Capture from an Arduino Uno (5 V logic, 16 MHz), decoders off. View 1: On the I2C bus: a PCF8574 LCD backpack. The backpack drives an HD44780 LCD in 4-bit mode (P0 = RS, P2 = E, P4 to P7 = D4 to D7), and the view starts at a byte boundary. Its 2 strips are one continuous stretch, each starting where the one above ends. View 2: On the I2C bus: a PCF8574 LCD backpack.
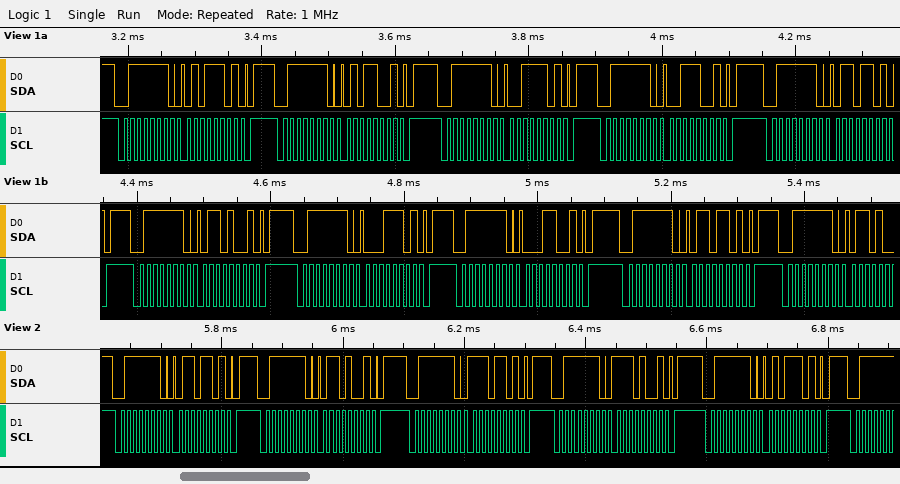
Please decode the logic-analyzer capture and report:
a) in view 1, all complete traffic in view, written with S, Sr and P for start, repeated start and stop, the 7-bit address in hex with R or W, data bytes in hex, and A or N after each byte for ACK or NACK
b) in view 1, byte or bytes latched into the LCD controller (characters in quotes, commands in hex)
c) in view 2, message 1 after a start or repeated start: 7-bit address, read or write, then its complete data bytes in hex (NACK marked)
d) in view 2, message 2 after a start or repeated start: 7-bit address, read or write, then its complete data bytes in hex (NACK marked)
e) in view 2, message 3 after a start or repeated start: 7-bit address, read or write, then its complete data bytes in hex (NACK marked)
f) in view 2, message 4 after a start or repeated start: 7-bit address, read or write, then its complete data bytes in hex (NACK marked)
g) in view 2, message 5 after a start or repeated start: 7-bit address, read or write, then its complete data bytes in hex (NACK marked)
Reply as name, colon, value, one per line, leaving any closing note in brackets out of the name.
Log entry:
in view 1, all complete traffic in view, written with S, Sr and P for start, repeated start and stop, the 7-bit address in hex with R or W, data bytes in hex, and A or N after each byte for ACK or NACK: S 3FW A 5D A P S 3FW A 59 A P S 3FW A 3D A P S 3FW A 39 A P S 3FW A 6D A P S 3FW A 69 A P S 3FW A 1D A P S 3FW A 19 A P S 3FW A 6D A P S 3FW A
in view 1, byte or bytes latched into the LCD controller: 'S' 'a'
in view 2, message 1 after a start or repeated start: 7-bit address, read or write, then its complete data bytes in hex: 0x3F write: 6D
in view 2, message 2 after a start or repeated start: 7-bit address, read or write, then its complete data bytes in hex: 0x3F write: 69
in view 2, message 3 after a start or repeated start: 7-bit address, read or write, then its complete data bytes in hex: 0x3F write: ED
in view 2, message 4 after a start or repeated start: 7-bit address, read or write, then its complete data bytes in hex: 0x3F write: E9
in view 2, message 5 after a start or repeated start: 7-bit address, read or write, then its complete data bytes in hex: 0x3F write: 5D
